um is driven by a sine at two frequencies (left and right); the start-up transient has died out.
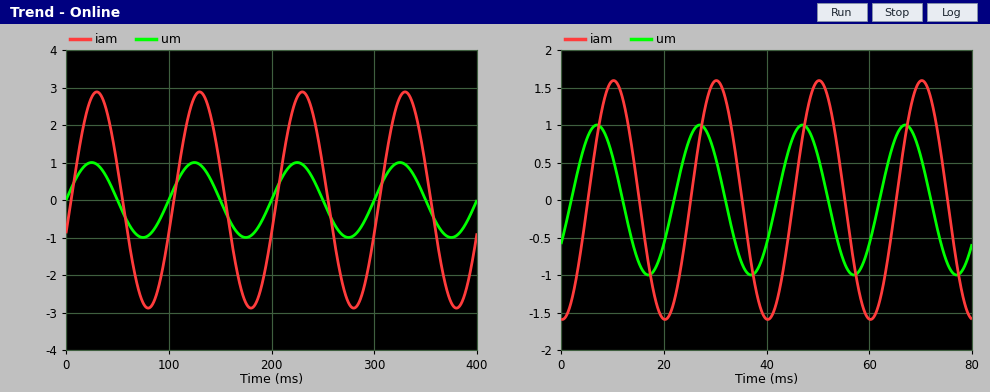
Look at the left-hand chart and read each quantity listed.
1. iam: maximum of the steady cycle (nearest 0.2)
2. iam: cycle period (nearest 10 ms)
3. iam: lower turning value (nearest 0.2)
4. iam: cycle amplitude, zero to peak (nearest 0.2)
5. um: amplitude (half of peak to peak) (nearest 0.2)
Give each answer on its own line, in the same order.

2.8
100 ms
-2.8
2.8
1.0
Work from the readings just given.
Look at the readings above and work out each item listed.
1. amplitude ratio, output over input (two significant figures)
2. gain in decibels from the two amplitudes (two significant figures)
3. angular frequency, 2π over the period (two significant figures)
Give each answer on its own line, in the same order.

2.8
8.9 dB
0.063 rad/ms
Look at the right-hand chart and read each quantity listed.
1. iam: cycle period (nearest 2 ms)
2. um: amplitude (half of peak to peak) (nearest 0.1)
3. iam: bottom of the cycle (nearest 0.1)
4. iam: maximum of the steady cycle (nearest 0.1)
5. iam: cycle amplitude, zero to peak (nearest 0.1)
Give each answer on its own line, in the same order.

20 ms
1.0
-1.6
1.6
1.6
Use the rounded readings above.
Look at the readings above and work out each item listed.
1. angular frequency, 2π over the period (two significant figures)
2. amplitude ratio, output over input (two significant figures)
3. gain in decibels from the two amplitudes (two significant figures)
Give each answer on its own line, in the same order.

0.31 rad/ms
1.6
4.1 dB
